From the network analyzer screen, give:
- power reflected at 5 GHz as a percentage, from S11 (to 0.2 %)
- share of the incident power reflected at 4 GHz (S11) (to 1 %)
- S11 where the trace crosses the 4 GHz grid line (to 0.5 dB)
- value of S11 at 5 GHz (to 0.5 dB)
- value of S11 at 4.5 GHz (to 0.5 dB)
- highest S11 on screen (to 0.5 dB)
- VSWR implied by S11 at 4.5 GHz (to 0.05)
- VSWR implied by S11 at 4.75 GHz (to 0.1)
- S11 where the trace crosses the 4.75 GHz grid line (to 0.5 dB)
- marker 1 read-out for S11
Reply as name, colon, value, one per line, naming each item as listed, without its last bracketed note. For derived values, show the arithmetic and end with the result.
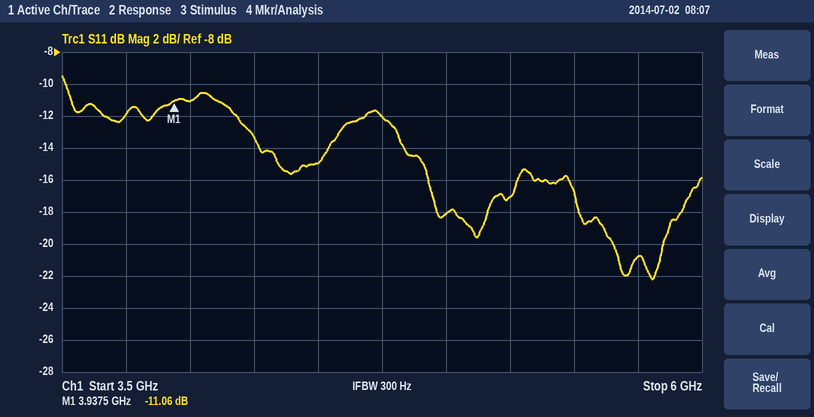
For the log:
power reflected at 5 GHz as a percentage, from S11: 10^(-18/10) ≈ 1.6 %
share of the incident power reflected at 4 GHz (S11): 10^(-11/10) ≈ 8 %
S11 where the trace crosses the 4 GHz grid line: -11.0 dB
value of S11 at 5 GHz: -18.0 dB
value of S11 at 4.5 GHz: -15.0 dB
highest S11 on screen: -9.5 dB
VSWR implied by S11 at 4.5 GHz: |Γ| = 10^(-15/20) = 0.1778; VSWR = (1 + 0.1778)/(1 − 0.1778) ≈ 1.43, so 1.45 to the nearest 0.05
VSWR implied by S11 at 4.75 GHz: |Γ| = 10^(-12/20) = 0.2512; VSWR = (1 + 0.2512)/(1 − 0.2512) ≈ 1.7
S11 where the trace crosses the 4.75 GHz grid line: -12.0 dB
marker 1 read-out for S11: -11.06 dB
